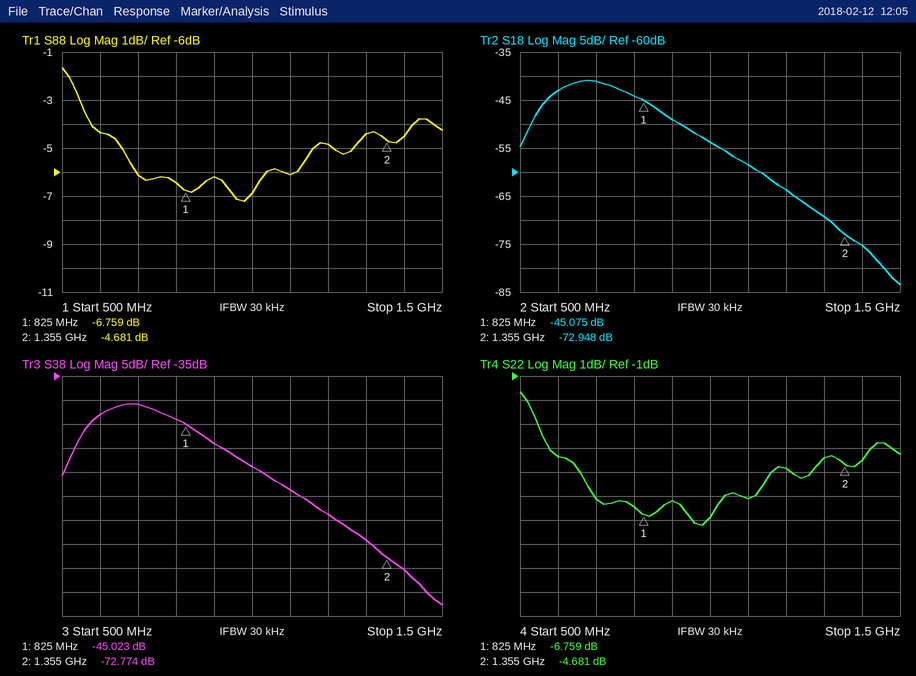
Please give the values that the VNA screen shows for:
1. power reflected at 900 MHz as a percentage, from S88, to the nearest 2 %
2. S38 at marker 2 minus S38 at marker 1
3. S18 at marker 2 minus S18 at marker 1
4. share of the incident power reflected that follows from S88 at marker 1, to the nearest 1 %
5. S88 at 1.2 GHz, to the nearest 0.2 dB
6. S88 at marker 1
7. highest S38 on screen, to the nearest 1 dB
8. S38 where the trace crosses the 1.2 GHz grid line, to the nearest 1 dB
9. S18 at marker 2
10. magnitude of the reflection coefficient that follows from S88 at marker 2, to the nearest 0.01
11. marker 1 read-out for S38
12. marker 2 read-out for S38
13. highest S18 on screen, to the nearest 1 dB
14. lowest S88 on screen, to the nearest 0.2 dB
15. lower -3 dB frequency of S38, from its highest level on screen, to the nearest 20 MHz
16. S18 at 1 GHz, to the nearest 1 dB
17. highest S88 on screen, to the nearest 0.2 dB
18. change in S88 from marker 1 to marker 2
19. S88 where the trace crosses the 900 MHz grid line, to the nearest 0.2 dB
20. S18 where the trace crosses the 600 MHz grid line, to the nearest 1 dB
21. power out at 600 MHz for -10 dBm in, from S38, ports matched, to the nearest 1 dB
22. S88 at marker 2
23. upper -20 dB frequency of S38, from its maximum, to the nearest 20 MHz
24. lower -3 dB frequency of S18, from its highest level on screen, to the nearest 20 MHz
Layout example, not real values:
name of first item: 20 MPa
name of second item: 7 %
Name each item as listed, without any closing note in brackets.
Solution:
power reflected at 900 MHz as a percentage, from S88, to the nearest 2 %: 24 %
S38 at marker 2 minus S38 at marker 1: -27.751 dB
S18 at marker 2 minus S18 at marker 1: -27.873 dB
share of the incident power reflected that follows from S88 at marker 1, to the nearest 1 %: 21 %
S88 at 1.2 GHz, to the nearest 0.2 dB: -4.8 dB
S88 at marker 1: -6.759 dB
highest S38 on screen, to the nearest 1 dB: -41 dB
S38 where the trace crosses the 1.2 GHz grid line, to the nearest 1 dB: -64 dB
S18 at marker 2: -72.948 dB
magnitude of the reflection coefficient that follows from S88 at marker 2, to the nearest 0.01: 0.58
marker 1 read-out for S38: -45.023 dB
marker 2 read-out for S38: -72.774 dB
highest S18 on screen, to the nearest 1 dB: -41 dB
lowest S88 on screen, to the nearest 0.2 dB: -7.2 dB
lower -3 dB frequency of S38, from its highest level on screen, to the nearest 20 MHz: 580 MHz
S18 at 1 GHz, to the nearest 1 dB: -54 dB
highest S88 on screen, to the nearest 0.2 dB: -1.6 dB
change in S88 from marker 1 to marker 2: 2.078 dB
S88 where the trace crosses the 900 MHz grid line, to the nearest 0.2 dB: -6.2 dB
S18 where the trace crosses the 600 MHz grid line, to the nearest 1 dB: -43 dB
power out at 600 MHz for -10 dBm in, from S38, ports matched, to the nearest 1 dB: -53 dBm
S88 at marker 2: -4.681 dB
upper -20 dB frequency of S38, from its maximum, to the nearest 20 MHz: 1.14 GHz
lower -3 dB frequency of S18, from its highest level on screen, to the nearest 20 MHz: 580 MHz
